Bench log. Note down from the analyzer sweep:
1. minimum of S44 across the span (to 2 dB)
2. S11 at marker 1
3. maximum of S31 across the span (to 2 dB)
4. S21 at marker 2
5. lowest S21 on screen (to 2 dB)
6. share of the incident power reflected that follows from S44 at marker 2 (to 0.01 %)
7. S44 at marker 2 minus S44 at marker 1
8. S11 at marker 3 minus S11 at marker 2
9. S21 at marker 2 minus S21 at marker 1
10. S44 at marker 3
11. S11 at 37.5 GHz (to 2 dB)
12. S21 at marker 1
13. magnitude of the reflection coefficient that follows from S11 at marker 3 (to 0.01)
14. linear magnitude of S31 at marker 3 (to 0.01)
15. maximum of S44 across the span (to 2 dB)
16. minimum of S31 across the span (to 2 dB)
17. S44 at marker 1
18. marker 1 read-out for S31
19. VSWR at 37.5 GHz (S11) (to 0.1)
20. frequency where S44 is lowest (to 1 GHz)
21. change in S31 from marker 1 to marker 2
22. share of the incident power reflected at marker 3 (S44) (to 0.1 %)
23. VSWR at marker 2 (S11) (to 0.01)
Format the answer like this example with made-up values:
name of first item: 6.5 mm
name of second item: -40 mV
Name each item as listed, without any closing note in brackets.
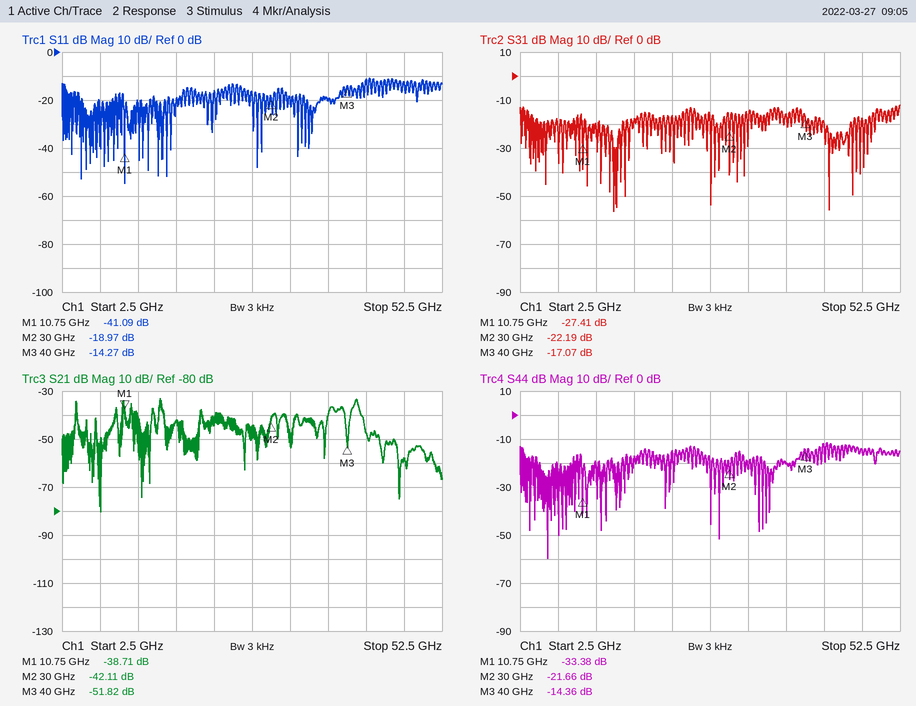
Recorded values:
minimum of S44 across the span: -60 dB
S11 at marker 1: -41.09 dB
maximum of S31 across the span: -12 dB
S21 at marker 2: -42.11 dB
lowest S21 on screen: -80 dB
share of the incident power reflected that follows from S44 at marker 2: 0.68 %
S44 at marker 2 minus S44 at marker 1: 11.72 dB
S11 at marker 3 minus S11 at marker 2: 4.70 dB
S21 at marker 2 minus S21 at marker 1: -3.40 dB
S44 at marker 3: -14.36 dB
S11 at 37.5 GHz: -20 dB
S21 at marker 1: -38.71 dB
magnitude of the reflection coefficient that follows from S11 at marker 3: 0.19
linear magnitude of S31 at marker 3: 0.14
maximum of S44 across the span: -12 dB
minimum of S31 across the span: -56 dB
S44 at marker 1: -33.38 dB
marker 1 read-out for S31: -27.41 dB
VSWR at 37.5 GHz (S11): 1.2
frequency where S44 is lowest: 6 GHz
change in S31 from marker 1 to marker 2: 5.22 dB
share of the incident power reflected at marker 3 (S44): 3.7 %
VSWR at marker 2 (S11): 1.25
